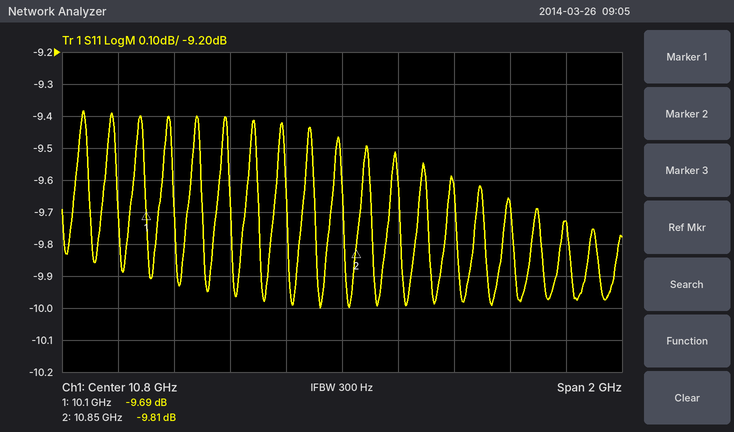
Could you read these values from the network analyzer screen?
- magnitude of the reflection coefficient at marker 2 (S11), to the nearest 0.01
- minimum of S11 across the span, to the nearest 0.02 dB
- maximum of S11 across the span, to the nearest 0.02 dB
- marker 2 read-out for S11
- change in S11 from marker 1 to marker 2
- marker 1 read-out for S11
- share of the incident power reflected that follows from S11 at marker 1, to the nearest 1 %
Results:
0.32
-10.00 dB
-9.38 dB
-9.81 dB
-0.12 dB
-9.69 dB
11 %
